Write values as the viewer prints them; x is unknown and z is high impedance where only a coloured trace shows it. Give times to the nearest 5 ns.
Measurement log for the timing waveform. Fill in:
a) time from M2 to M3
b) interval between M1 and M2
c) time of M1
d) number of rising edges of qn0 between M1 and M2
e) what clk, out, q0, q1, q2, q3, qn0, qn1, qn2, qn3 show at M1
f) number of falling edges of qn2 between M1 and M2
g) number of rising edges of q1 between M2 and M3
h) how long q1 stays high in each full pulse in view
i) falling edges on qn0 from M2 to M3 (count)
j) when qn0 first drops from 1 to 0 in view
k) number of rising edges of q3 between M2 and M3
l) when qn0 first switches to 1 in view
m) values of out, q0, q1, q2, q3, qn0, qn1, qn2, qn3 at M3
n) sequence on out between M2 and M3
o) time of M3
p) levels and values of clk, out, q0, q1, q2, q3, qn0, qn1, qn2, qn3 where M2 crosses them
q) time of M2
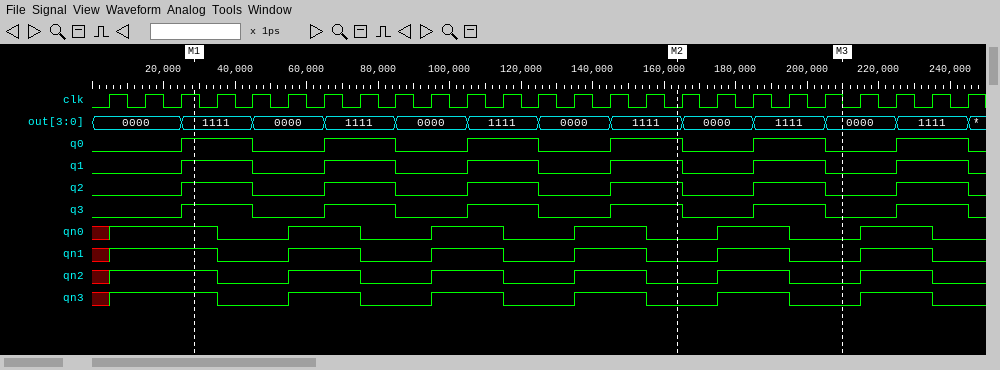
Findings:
45 ns
135 ns
30 ns
3
clk=1, out=1111, q0=1, q1=1, q2=1, q3=1, qn0=1, qn1=1, qn2=1, qn3=1
4
1
20 ns, 20 ns, 20 ns, 20 ns, 20 ns, 20 ns
1
35 ns
1
5 ns
out=0000, q0=0, q1=0, q2=0, q3=0, qn0=0, qn1=0, qn2=0, qn3=0
1111, 0000, 1111, 0000
210 ns
clk=0, out=1111, q0=1, q1=1, q2=1, q3=1, qn0=0, qn1=0, qn2=0, qn3=0
165 ns
